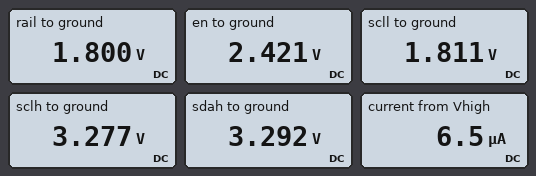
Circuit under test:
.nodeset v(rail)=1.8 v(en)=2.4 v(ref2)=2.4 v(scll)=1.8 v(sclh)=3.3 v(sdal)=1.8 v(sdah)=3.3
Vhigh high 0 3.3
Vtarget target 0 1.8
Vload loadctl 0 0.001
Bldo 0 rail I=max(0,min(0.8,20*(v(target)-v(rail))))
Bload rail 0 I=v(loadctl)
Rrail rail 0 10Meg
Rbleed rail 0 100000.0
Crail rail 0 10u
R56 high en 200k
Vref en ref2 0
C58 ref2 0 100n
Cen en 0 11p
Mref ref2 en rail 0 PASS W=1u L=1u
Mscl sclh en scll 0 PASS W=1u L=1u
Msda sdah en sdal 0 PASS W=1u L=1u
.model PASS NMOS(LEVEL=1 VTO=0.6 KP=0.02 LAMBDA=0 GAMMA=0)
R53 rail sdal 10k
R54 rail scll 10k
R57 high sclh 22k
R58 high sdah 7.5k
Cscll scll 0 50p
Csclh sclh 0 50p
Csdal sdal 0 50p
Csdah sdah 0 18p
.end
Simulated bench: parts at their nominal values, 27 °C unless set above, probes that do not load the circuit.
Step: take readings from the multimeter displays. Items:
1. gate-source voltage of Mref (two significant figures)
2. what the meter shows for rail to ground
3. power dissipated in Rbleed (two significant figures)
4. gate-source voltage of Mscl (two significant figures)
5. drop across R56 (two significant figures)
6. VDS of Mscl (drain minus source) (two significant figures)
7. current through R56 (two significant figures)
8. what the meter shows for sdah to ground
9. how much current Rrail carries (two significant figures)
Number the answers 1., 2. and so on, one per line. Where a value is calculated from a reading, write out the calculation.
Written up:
1. 2.421 V - 1.8 V = 620 mV
2. 1.800 V
3. (1.8 V)^2 / 100 kΩ = 32 µW
4. 2.421 V - 1.811 V = 610 mV
5. 3.3 V - 2.421 V = 880 mV
6. 3.277 V - 1.811 V = 1.5 V
7. (3.3 V - 2.421 V) / 200 kΩ = 4.4 µA
8. 3.292 V
9. (1.8 V) / 10 MΩ = 180 nA
